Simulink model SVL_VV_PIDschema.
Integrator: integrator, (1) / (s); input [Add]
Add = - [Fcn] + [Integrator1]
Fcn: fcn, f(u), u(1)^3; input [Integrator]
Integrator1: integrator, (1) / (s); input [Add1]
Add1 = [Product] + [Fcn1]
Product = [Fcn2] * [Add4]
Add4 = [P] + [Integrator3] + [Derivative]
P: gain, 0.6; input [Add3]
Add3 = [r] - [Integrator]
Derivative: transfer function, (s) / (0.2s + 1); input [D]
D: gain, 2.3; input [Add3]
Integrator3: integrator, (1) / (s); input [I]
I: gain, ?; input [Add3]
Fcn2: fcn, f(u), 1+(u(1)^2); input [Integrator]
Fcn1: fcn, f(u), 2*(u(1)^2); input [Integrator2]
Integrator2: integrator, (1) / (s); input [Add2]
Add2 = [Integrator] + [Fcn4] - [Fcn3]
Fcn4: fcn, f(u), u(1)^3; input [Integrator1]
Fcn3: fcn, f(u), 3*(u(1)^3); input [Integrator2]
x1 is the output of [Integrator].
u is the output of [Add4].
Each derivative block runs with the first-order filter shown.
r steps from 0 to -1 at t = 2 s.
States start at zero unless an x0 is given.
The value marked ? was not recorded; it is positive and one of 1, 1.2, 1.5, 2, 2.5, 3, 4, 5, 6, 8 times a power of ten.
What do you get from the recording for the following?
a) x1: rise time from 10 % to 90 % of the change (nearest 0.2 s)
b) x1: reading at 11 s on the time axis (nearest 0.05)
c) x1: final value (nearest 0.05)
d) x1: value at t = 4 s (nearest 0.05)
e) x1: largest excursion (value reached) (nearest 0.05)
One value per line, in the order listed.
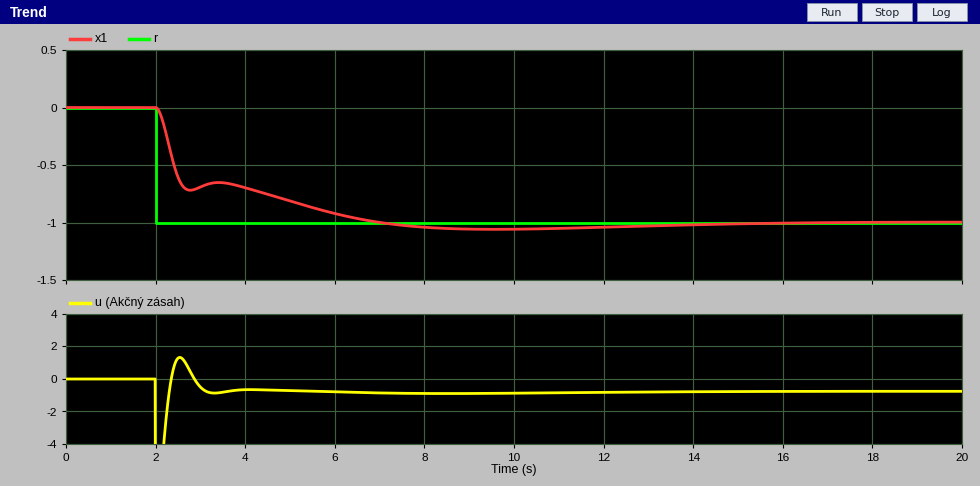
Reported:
3.6 s
-1.05
-1.00
-0.70
-1.05
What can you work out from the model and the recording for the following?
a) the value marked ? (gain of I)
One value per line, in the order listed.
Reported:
0.8
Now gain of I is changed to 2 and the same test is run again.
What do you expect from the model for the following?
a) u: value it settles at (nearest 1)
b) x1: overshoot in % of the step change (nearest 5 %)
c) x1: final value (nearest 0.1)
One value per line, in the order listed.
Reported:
-1
10 %
-1.0
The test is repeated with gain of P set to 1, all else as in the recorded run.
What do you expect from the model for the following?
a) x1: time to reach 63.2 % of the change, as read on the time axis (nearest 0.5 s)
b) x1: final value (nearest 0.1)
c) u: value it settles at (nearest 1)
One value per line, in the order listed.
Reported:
2.5 s
-1.0
-1
